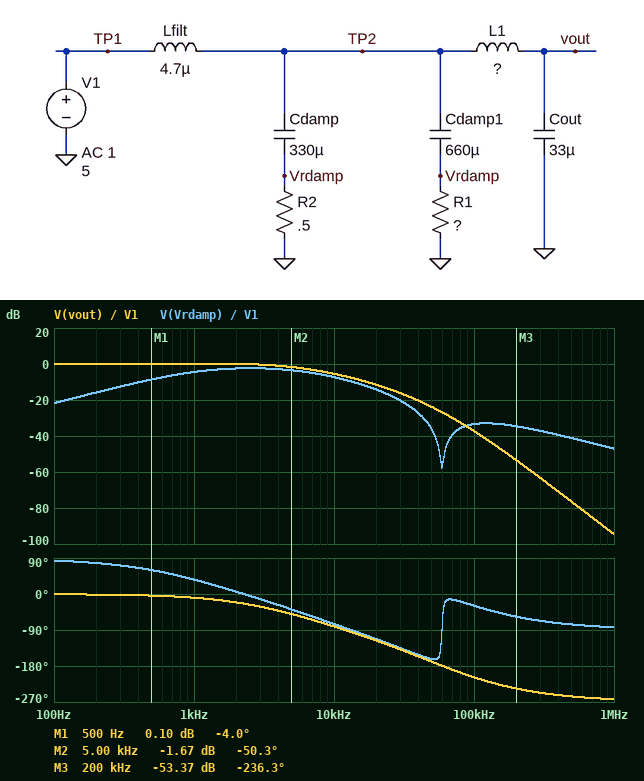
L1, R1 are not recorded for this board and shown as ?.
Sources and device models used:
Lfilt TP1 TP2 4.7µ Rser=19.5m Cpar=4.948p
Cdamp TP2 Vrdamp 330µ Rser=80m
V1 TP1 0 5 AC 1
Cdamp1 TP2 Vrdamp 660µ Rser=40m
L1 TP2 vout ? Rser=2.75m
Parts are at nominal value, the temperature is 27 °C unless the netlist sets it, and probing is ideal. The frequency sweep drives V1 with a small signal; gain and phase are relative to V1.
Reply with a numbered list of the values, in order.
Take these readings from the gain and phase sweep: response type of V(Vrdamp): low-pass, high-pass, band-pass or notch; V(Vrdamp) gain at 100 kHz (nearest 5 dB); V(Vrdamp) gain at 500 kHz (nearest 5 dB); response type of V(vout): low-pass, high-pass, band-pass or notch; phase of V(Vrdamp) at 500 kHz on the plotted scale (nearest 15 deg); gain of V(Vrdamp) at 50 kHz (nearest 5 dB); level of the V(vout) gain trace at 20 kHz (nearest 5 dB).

1. band-pass
2. -35 dB
3. -40 dB
4. low-pass
5. -75 deg
6. -35 dB
7. -10 dB
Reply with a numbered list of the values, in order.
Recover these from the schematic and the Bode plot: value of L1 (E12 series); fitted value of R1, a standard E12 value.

1. 220 nH
2. 0.18 Ω
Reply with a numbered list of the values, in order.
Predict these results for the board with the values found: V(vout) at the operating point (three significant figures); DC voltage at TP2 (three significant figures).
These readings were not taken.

1. 5.00 V
2. 5.00 V
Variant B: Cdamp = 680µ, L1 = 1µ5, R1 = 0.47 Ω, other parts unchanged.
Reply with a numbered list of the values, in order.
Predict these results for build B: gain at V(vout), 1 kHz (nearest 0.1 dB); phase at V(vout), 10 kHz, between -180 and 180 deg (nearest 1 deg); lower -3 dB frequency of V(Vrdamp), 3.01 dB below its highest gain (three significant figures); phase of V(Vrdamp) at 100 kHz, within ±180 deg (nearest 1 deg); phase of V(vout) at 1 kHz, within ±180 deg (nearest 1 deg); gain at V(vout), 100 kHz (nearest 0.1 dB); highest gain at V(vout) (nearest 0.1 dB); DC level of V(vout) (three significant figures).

1. -0.2 dB
2. -78 deg
3. 425 Hz
4. -68 deg
5. -7 deg
6. -46.8 dB
7. 0.5 dB
8. 5.00 V
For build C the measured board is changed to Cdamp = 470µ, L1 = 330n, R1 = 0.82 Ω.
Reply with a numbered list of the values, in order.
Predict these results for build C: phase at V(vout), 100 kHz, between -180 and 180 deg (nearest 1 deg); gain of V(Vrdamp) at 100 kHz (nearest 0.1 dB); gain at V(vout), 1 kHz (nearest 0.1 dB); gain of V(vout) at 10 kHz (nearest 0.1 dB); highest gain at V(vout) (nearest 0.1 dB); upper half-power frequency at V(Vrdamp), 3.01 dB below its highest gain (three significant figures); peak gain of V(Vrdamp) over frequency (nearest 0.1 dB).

1. 156 deg
2. -27.4 dB
3. -0.1 dB
4. 0.4 dB
5. 0.6 dB
6. 14.2 kHz
7. -0.4 dB
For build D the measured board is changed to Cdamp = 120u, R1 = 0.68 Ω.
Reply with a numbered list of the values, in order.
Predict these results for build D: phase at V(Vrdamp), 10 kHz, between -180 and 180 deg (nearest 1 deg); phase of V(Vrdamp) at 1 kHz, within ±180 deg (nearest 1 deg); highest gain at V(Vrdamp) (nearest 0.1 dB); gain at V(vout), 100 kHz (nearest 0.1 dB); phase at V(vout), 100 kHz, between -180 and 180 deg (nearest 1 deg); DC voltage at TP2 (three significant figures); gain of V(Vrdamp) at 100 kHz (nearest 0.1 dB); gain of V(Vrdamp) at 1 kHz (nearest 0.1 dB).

1. -65 deg
2. 27 deg
3. -0.6 dB
4. -36.4 dB
5. 165 deg
6. 5.00 V
7. -31.7 dB
8. -2.4 dB
